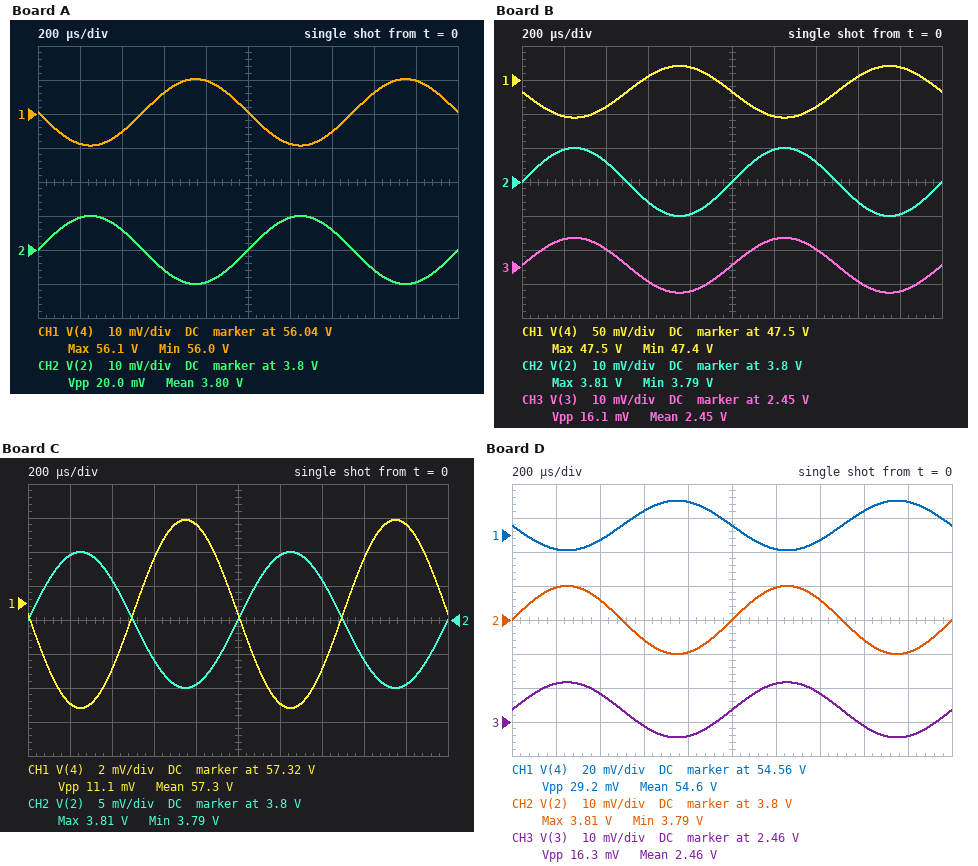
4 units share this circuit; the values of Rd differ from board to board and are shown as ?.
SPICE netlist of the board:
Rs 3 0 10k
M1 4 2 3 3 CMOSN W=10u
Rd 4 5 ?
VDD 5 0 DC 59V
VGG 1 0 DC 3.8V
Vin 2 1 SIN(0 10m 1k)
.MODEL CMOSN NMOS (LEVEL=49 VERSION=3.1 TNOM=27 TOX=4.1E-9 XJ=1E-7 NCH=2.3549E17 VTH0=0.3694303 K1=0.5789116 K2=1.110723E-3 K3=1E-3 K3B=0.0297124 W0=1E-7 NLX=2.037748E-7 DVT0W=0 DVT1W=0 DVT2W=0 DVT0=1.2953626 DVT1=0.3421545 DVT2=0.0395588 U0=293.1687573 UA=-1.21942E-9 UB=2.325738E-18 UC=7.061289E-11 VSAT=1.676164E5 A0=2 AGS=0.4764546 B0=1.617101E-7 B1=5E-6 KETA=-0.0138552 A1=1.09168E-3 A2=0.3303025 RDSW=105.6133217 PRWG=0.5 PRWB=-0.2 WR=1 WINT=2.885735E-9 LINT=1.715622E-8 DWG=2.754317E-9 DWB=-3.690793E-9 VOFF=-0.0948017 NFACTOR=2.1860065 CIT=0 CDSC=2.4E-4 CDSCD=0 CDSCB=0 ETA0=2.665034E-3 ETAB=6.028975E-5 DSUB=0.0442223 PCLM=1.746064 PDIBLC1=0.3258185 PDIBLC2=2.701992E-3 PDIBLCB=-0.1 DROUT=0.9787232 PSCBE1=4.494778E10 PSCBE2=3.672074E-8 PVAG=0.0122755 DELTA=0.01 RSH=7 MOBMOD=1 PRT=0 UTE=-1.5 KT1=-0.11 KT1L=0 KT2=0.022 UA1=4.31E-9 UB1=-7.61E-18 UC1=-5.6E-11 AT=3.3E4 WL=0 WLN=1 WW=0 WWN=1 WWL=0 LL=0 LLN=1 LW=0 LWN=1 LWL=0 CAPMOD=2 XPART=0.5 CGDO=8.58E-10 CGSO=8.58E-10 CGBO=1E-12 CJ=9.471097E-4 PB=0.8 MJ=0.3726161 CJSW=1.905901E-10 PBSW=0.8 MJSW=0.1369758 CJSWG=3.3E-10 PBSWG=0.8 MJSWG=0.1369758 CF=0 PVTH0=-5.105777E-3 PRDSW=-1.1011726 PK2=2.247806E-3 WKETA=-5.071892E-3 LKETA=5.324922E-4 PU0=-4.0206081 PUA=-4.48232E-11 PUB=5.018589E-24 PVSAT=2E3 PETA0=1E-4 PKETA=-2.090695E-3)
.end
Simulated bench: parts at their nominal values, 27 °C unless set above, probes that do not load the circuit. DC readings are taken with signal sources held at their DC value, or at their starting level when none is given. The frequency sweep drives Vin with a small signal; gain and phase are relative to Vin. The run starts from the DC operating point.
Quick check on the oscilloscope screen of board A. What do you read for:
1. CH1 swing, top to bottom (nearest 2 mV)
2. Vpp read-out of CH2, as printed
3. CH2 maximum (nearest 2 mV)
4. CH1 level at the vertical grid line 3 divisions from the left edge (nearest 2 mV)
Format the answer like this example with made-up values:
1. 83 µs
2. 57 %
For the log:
1. 20 mV
2. 20.0 mV
3. 3.810 V
4. 56.046 V
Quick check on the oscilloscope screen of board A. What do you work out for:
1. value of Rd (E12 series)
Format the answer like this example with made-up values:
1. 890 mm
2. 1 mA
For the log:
1. 12 kΩ
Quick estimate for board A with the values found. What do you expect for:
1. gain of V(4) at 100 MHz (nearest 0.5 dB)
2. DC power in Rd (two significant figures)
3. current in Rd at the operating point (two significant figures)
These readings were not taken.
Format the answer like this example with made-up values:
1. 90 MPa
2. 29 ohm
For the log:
1. 0 dB
2. 730 µW
3. 250 µA
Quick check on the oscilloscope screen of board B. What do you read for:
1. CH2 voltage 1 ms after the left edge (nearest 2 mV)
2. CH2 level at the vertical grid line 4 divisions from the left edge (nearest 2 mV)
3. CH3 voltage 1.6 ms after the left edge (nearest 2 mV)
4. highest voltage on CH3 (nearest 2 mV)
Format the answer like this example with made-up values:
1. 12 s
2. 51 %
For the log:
1. 3.800 V
2. 3.790 V
3. 2.446 V
4. 2.458 V
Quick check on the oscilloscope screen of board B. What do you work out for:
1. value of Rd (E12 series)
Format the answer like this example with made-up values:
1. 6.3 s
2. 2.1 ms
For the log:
1. 47 kΩ
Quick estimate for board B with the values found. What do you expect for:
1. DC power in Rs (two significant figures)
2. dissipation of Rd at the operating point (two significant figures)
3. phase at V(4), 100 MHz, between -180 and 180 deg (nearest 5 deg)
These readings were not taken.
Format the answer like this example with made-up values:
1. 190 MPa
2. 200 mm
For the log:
1. 600 µW
2. 2.8 mW
3. 135 deg
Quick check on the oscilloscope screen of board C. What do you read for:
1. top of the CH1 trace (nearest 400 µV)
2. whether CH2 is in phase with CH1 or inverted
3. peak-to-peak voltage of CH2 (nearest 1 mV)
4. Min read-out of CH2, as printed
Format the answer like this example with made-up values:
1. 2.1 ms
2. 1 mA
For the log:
1. 57.3268 V
2. inverted
3. 20 mV
4. 3.79 V
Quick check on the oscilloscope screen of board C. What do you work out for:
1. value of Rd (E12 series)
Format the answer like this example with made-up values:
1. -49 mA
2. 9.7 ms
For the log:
1. 6.8 kΩ
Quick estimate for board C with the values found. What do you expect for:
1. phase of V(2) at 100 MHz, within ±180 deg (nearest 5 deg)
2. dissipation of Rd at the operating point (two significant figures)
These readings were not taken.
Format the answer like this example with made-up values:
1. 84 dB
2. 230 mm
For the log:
1. 0 deg
2. 410 µW
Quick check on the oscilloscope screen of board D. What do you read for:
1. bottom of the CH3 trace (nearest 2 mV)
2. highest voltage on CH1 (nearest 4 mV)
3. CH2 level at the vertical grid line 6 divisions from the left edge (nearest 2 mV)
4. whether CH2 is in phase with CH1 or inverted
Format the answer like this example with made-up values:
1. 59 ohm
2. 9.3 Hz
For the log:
1. 2.456 V
2. 54.580 V
3. 3.810 V
4. inverted
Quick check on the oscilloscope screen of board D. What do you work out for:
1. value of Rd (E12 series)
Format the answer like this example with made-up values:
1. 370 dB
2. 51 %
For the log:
1. 18 kΩ
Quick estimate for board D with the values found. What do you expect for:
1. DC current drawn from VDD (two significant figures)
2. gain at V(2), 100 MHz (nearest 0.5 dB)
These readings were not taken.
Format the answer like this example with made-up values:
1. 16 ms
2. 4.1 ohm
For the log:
1. 250 µA
2. 0 dB
